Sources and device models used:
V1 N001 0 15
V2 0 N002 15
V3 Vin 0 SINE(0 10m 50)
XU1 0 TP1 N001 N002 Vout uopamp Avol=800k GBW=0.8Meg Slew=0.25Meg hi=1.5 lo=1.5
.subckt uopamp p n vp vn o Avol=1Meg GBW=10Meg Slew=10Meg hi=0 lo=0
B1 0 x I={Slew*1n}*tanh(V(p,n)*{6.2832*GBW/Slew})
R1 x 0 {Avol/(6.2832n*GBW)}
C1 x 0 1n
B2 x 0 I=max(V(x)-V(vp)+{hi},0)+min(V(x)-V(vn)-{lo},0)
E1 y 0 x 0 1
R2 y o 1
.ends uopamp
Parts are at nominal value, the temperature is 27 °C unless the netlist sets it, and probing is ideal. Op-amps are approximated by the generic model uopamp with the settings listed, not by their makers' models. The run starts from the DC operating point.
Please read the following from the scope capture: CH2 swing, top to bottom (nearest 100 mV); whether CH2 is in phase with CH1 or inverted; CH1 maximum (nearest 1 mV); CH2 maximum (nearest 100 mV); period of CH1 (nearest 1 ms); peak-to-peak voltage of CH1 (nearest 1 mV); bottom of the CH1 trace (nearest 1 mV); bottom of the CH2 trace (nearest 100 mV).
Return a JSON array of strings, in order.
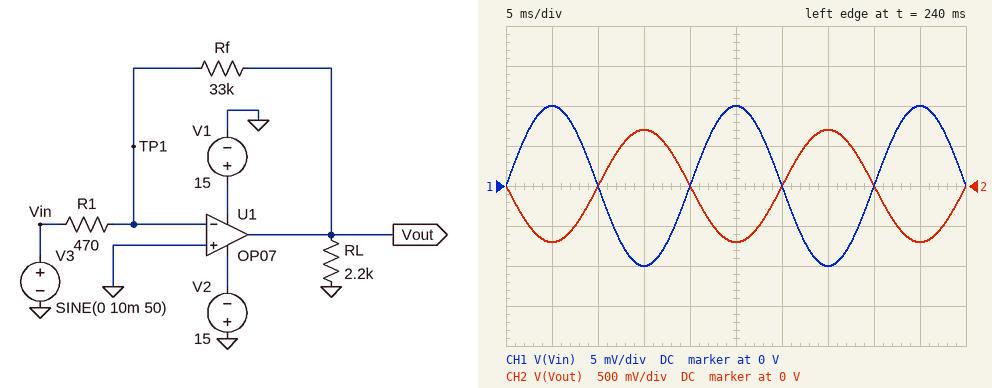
["1.4 V", "inverted", "10 mV", "700 mV", "20 ms", "20 mV", "-10 mV", "-700 mV"]
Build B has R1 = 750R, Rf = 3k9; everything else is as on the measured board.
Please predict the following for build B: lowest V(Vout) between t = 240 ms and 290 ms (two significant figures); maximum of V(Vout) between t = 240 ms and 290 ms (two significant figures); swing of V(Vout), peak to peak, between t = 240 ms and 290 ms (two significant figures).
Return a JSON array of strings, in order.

["-52 mV", "52 mV", "100 mV"]
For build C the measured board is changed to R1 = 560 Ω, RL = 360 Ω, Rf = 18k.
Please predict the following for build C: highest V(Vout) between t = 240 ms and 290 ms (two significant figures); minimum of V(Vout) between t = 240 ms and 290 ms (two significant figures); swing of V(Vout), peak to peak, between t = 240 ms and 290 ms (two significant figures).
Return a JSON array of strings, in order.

["320 mV", "-320 mV", "640 mV"]
